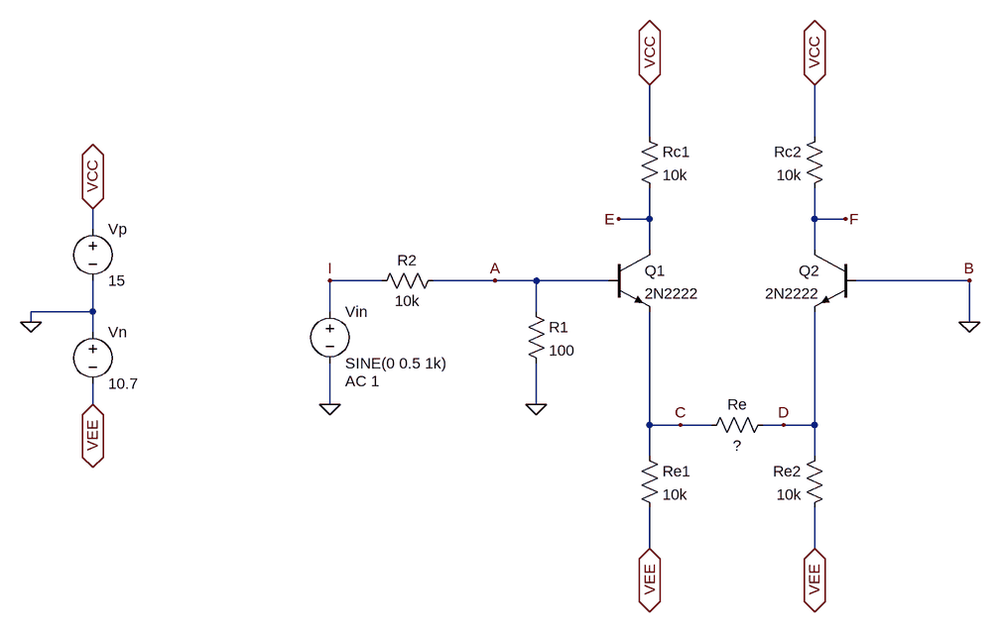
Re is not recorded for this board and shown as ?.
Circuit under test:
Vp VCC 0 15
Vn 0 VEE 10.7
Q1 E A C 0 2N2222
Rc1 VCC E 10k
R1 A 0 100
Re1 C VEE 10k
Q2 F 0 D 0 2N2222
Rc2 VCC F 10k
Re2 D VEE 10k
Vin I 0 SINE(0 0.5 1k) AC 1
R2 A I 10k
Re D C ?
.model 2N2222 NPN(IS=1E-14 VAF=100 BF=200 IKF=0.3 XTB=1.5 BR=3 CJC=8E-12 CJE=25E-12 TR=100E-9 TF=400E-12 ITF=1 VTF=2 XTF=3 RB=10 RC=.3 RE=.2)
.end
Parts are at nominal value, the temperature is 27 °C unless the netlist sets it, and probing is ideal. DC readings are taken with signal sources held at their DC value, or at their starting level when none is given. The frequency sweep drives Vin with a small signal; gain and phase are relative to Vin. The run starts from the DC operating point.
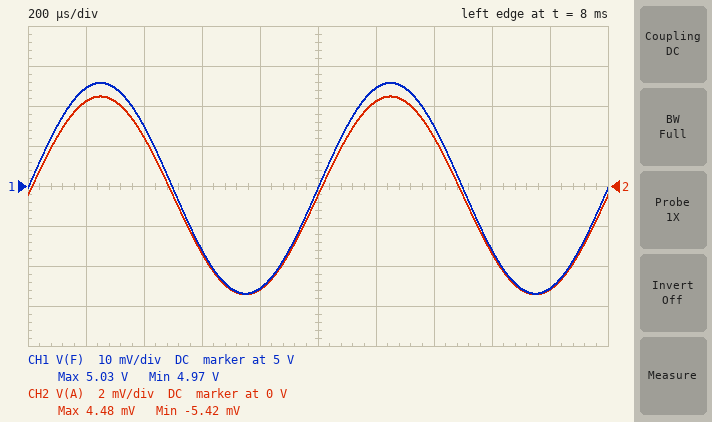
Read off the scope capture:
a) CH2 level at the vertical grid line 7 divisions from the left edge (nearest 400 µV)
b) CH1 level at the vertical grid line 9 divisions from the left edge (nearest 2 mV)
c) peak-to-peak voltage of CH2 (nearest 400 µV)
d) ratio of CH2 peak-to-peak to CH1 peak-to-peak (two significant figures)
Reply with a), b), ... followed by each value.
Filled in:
a) 2.4 mV
b) 4.974 V
c) 10.0 mV
d) 0.19
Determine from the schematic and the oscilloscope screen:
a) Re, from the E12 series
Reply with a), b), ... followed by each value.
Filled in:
a) 1.8 kΩ
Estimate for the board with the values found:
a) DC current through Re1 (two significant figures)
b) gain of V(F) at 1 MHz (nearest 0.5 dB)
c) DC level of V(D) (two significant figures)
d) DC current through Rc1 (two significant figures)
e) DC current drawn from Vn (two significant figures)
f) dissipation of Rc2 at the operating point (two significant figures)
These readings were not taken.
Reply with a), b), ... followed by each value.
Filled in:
a) 1.0 mA
b) -26.0 dB
c) -650 mV
d) 1.0 mA
e) 2.0 mA
f) 10 mW
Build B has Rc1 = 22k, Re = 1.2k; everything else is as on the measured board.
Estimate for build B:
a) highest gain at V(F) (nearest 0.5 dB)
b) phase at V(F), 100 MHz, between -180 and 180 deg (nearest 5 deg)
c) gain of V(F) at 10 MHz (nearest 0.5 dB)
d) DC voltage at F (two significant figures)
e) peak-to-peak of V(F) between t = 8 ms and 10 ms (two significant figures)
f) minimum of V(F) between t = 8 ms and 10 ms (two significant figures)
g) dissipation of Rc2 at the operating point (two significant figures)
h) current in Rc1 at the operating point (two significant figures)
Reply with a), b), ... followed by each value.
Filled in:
a) -23.0 dB
b) -125 deg
c) -32.0 dB
d) 4.7 V
e) 69 mV
f) 4.6 V
g) 11 mW
h) 710 µA
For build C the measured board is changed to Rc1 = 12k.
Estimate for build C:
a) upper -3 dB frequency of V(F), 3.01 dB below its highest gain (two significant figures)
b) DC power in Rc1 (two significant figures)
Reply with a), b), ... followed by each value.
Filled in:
a) 3.5 MHz
b) 12 mW
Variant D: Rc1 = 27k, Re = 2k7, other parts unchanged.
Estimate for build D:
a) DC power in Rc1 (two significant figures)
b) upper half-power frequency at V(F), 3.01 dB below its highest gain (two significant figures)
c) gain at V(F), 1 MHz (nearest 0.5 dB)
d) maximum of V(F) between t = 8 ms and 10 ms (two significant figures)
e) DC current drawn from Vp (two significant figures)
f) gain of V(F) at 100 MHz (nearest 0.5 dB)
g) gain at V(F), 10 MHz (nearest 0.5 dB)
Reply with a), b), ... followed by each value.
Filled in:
a) 9.1 mW
b) 3.9 MHz
c) -29.5 dB
d) 4.8 V
e) 1.6 mA
f) -60.5 dB
g) -38.5 dB
